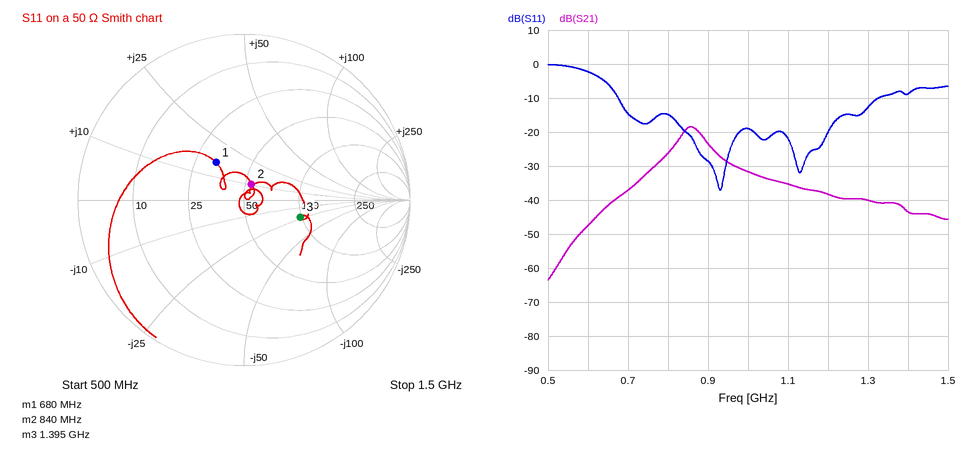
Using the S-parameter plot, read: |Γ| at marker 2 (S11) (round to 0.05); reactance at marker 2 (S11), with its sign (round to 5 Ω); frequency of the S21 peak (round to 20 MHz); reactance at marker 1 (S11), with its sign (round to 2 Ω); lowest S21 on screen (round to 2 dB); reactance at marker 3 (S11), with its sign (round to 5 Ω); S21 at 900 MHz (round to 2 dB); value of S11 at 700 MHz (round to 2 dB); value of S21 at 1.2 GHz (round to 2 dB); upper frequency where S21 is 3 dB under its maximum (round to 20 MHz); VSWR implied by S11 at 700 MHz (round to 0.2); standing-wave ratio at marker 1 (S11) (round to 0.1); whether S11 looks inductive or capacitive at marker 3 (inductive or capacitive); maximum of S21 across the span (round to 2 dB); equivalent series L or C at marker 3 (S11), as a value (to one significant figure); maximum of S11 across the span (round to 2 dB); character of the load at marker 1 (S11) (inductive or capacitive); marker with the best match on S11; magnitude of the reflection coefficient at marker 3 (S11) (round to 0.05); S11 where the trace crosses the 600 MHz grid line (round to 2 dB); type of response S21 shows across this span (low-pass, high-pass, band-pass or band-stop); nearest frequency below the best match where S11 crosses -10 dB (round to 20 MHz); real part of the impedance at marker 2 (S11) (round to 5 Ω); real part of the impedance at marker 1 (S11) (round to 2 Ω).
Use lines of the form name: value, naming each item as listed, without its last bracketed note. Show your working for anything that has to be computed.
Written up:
|Γ| at marker 2 (S11): 0.10
reactance at marker 2 (S11), with its sign: +10 Ω
frequency of the S21 peak: 860 MHz
reactance at marker 1 (S11), with its sign: +16 Ω
lowest S21 on screen: -64 dB
reactance at marker 3 (S11), with its sign: -25 Ω
S21 at 900 MHz: -24 dB
value of S11 at 700 MHz: -14 dB
value of S21 at 1.2 GHz: -38 dB
upper frequency where S21 is 3 dB under its maximum: 880 MHz
VSWR implied by S11 at 700 MHz: |Γ| = 10^(-14/20) = 0.1995; VSWR = (1 + 0.1995)/(1 − 0.1995) ≈ 1.50, so 1.4 to the nearest 0.2
standing-wave ratio at marker 1 (S11): 1.8
whether S11 looks inductive or capacitive at marker 3: capacitive
maximum of S21 across the span: -18 dB
equivalent series L or C at marker 3 (S11), as a value: C = 1/(2π × 1.395 GHz × 25 Ω) ≈ 5 pF
maximum of S11 across the span: 0 dB
character of the load at marker 1 (S11): inductive
marker with the best match on S11: marker 2
magnitude of the reflection coefficient at marker 3 (S11): 0.35
S11 where the trace crosses the 600 MHz grid line: -2 dB
type of response S21 shows across this span: band-pass
nearest frequency below the best match where S11 crosses -10 dB: 680 MHz
real part of the impedance at marker 2 (S11): 55 Ω
real part of the impedance at marker 1 (S11): 32 Ω
